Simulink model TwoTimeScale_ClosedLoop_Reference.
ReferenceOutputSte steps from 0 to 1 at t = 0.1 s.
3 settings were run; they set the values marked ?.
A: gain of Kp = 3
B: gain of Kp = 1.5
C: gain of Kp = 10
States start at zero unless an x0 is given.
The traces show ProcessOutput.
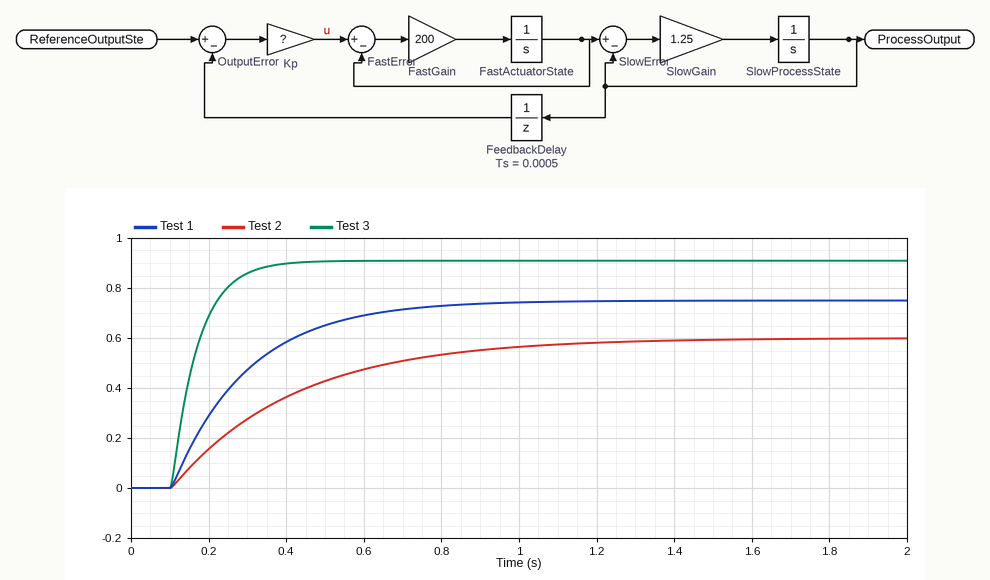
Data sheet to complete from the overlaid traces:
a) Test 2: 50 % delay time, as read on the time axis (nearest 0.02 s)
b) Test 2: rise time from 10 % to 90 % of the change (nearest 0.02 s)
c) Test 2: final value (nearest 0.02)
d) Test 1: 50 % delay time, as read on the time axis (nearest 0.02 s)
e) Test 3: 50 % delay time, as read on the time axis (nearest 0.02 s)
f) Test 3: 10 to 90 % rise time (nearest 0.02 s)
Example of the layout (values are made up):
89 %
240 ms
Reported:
0.32 s
0.70 s
0.60
0.24 s
0.16 s
0.14 s
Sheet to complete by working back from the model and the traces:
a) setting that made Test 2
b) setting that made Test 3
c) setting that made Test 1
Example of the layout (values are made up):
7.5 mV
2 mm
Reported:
B
C
A
